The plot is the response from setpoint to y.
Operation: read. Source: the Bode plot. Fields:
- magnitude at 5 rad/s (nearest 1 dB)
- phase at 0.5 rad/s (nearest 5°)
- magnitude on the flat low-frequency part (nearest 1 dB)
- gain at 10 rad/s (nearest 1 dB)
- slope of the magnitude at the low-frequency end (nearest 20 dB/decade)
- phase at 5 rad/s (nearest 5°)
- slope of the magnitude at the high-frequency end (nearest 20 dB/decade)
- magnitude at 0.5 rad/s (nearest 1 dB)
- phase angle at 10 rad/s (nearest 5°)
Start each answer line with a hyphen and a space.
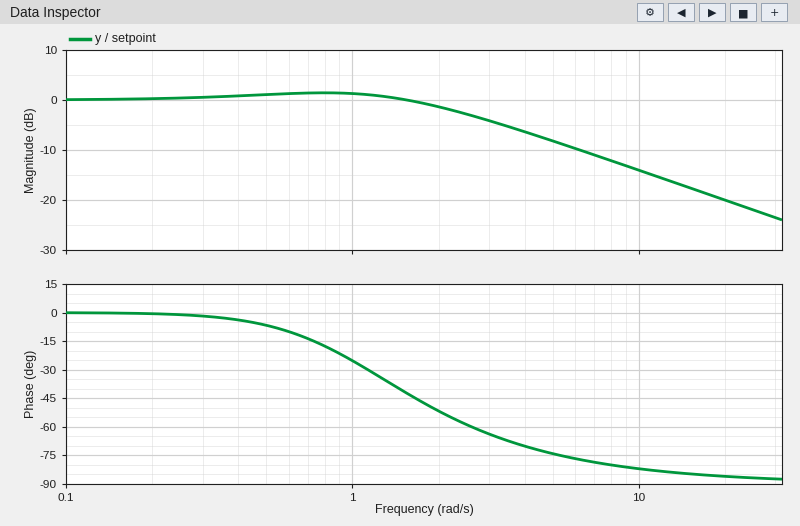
- -8 dB
- -5°
- 0 dB
- -14 dB
- 0 dB/decade
- -75°
- -20 dB/decade
- 1 dB
- -80°
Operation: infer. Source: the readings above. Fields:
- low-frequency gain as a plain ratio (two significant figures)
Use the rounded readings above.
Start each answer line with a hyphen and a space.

- 1.0
